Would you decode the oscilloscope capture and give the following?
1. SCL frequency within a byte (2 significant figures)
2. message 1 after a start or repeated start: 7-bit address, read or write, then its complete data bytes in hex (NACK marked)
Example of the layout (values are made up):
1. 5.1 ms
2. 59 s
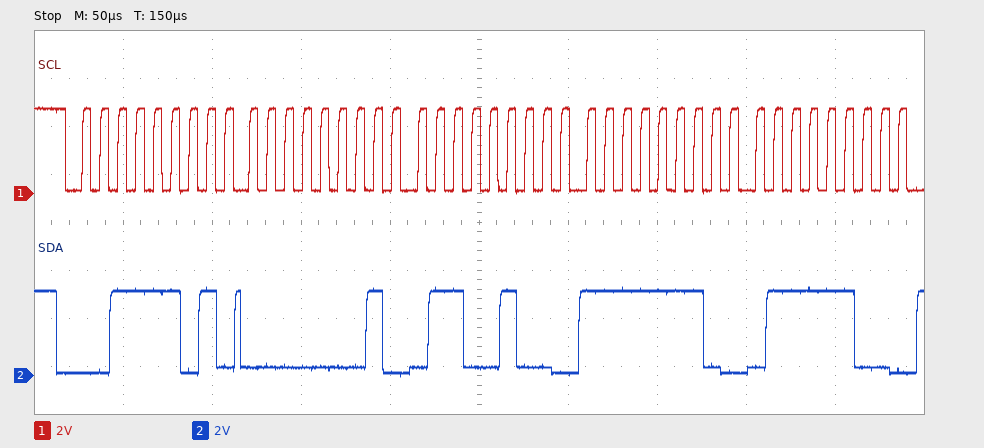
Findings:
1. 100 kHz
2. 0x1E read: 01 64 FE 7C
